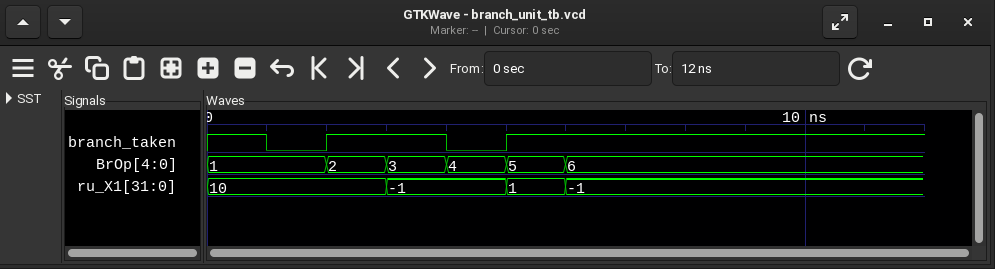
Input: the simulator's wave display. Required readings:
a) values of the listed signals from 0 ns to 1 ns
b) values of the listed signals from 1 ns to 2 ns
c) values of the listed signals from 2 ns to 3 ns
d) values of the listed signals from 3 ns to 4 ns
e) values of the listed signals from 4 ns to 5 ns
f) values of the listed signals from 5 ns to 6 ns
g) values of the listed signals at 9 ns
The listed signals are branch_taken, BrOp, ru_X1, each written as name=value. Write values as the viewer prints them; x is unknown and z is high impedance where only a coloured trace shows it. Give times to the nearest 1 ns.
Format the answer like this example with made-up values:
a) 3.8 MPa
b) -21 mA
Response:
a) branch_taken=1, BrOp=1, ru_X1=10
b) branch_taken=0, BrOp=1, ru_X1=10
c) branch_taken=1, BrOp=2, ru_X1=10
d) branch_taken=1, BrOp=3, ru_X1=-1
e) branch_taken=0, BrOp=4, ru_X1=-1
f) branch_taken=1, BrOp=5, ru_X1=1
g) branch_taken=1, BrOp=6, ru_X1=-1
